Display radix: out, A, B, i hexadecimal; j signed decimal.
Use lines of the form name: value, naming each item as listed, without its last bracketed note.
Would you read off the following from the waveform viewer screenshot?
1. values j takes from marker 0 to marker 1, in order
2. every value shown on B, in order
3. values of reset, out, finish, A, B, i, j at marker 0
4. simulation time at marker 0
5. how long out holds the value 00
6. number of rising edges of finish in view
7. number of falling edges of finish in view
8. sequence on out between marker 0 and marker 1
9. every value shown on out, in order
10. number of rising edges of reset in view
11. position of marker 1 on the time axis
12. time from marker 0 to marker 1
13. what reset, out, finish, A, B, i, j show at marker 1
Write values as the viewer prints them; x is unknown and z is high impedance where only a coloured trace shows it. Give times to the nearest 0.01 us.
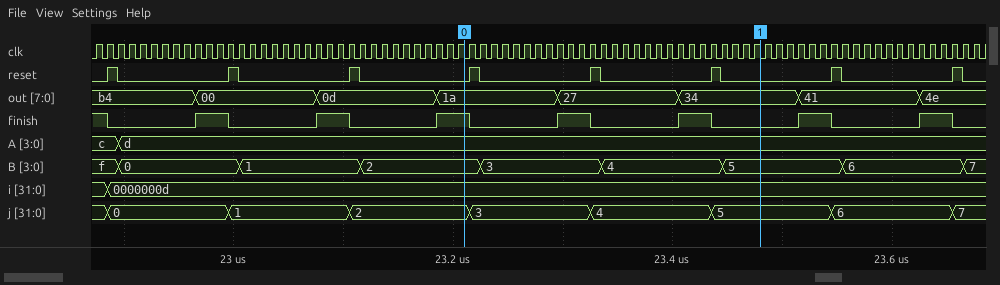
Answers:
values j takes from marker 0 to marker 1, in order: 2, 3, 4, 5
every value shown on B, in order: f, 0, 1, 2, 3, 4, 5, 6, 7
values of reset, out, finish, A, B, i, j at marker 0: reset=0, out=1a, finish=1, A=d, B=2, i=0000000d, j=2
simulation time at marker 0: 23.21 us
how long out holds the value 00: 0.11 us
number of rising edges of finish in view: 7
number of falling edges of finish in view: 8
sequence on out between marker 0 and marker 1: 1a, 27, 34
every value shown on out, in order: b4, 00, 0d, 1a, 27, 34, 41, 4e
number of rising edges of reset in view: 8
position of marker 1 on the time axis: 23.48 us
time from marker 0 to marker 1: 0.27 us
what reset, out, finish, A, B, i, j show at marker 1: reset=0, out=34, finish=0, A=d, B=5, i=0000000d, j=5
